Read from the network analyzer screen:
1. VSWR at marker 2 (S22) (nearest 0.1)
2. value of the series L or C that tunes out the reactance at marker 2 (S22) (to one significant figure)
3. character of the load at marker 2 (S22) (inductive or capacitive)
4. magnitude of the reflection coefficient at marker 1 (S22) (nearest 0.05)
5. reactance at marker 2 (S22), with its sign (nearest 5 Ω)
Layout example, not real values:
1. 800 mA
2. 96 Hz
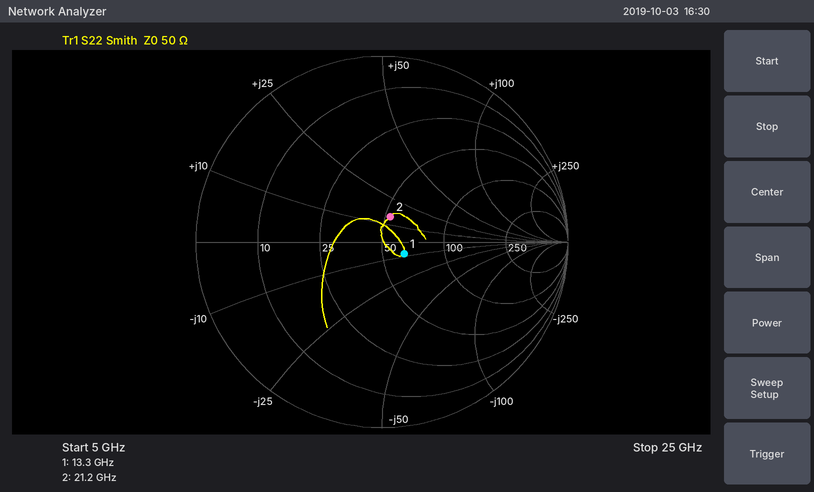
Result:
1. 1.3
2. 500 fF
3. inductive
4. 0.15
5. +15 Ω
